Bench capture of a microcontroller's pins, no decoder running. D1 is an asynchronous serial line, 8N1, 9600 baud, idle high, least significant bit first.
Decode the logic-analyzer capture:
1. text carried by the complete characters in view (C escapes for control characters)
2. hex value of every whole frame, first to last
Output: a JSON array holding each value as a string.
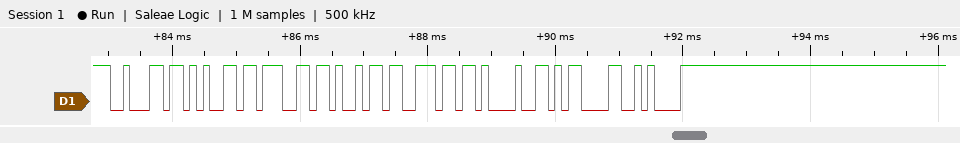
["\"begin!\\r\\n\"", "0x62 0x65 0x67 0x69 0x6E 0x21 0x0D 0x0A"]
